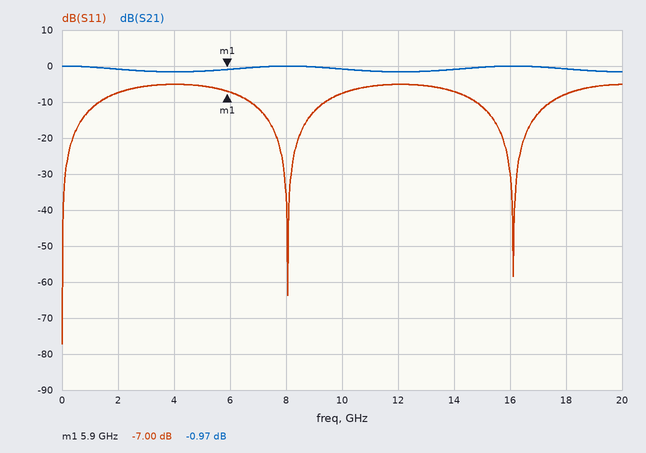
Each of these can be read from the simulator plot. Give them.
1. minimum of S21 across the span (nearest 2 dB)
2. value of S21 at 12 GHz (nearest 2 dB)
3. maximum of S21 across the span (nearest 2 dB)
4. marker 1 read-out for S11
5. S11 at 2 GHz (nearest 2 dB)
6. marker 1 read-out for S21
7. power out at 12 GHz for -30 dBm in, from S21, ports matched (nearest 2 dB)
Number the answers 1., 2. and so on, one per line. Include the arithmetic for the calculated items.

1. -2 dB
2. -2 dB
3. 0 dB
4. -7.00 dB
5. -8 dB
6. -0.97 dB
7. -30 dBm + (-2 dB) = -32 dBm
